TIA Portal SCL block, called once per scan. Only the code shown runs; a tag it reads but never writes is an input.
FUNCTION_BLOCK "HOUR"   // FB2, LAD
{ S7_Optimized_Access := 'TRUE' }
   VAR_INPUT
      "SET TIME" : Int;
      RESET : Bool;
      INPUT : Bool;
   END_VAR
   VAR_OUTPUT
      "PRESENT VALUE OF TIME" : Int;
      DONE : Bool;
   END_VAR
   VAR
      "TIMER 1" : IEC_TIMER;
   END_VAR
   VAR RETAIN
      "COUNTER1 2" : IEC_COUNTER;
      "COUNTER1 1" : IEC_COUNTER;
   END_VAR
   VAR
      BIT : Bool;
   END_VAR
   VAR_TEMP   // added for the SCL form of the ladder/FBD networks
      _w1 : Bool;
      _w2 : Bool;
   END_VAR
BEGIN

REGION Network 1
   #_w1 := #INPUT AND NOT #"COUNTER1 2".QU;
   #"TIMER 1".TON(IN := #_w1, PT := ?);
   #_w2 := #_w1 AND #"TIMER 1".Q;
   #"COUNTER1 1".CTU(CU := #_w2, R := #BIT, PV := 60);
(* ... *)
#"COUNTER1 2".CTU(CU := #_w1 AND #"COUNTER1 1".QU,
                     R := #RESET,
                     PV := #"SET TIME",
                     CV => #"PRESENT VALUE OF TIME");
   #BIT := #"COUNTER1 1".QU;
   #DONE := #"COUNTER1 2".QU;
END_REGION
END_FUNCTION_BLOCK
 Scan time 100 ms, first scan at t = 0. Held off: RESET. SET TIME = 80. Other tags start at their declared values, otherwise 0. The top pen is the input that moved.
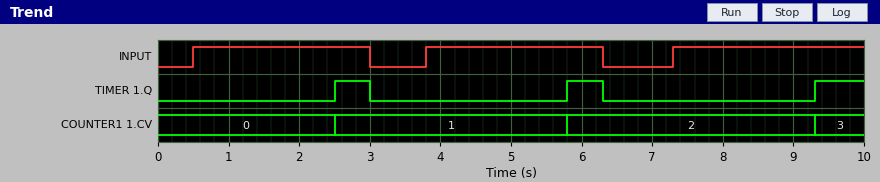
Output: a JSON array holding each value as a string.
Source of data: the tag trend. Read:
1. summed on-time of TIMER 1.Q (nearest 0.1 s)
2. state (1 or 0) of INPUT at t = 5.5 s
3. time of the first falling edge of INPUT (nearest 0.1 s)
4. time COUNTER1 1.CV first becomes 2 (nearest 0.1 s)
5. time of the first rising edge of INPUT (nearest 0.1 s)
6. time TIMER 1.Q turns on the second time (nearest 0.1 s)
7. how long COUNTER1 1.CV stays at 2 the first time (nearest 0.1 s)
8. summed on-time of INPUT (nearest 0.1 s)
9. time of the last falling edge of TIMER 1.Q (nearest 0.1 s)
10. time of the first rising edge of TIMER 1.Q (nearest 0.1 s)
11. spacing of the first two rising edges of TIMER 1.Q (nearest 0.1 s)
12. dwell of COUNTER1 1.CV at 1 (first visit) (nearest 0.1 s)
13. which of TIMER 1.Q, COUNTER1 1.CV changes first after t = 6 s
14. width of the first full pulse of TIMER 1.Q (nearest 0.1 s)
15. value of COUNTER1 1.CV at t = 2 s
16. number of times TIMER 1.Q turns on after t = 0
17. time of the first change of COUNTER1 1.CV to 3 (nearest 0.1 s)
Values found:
["1.7 s", "1", "3.0 s", "5.8 s", "0.5 s", "5.8 s", "3.5 s", "7.7 s", "6.3 s", "2.5 s", "3.3 s", "3.3 s", "TIMER 1.Q", "0.5 s", "0", "3", "9.3 s"]
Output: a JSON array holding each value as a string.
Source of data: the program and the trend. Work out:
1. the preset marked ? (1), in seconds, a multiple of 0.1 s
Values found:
["2.0 s"]
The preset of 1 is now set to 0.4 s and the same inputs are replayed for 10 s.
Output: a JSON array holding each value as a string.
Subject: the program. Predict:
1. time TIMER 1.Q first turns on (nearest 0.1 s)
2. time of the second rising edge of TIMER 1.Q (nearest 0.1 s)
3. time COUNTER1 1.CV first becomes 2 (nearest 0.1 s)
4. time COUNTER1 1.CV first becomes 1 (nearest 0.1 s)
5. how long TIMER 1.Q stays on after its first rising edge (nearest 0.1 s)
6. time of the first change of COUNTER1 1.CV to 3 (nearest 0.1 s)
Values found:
["0.9 s", "4.2 s", "4.2 s", "0.9 s", "2.1 s", "7.7 s"]
